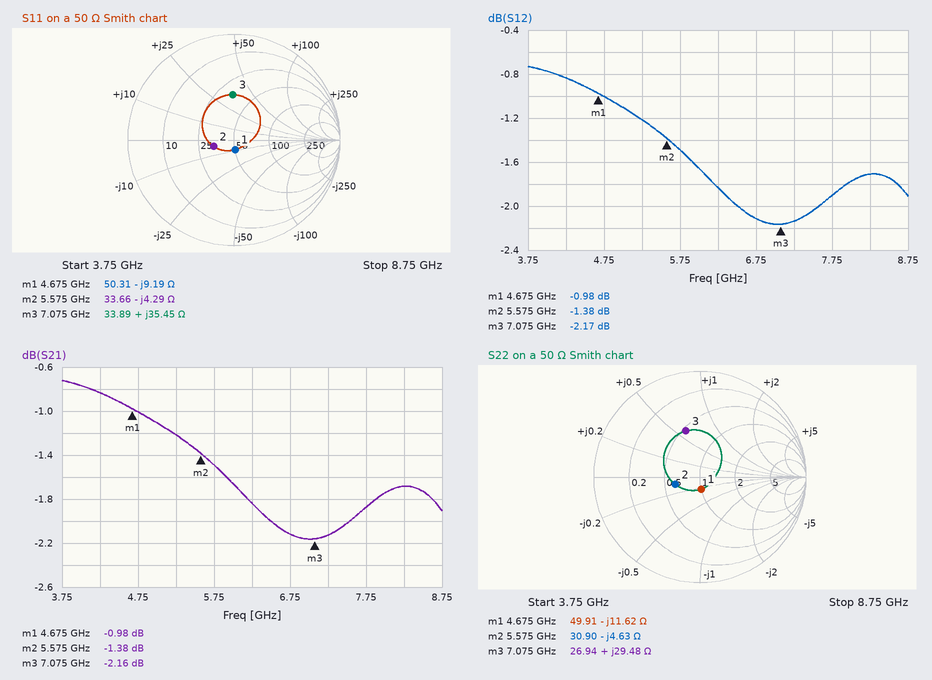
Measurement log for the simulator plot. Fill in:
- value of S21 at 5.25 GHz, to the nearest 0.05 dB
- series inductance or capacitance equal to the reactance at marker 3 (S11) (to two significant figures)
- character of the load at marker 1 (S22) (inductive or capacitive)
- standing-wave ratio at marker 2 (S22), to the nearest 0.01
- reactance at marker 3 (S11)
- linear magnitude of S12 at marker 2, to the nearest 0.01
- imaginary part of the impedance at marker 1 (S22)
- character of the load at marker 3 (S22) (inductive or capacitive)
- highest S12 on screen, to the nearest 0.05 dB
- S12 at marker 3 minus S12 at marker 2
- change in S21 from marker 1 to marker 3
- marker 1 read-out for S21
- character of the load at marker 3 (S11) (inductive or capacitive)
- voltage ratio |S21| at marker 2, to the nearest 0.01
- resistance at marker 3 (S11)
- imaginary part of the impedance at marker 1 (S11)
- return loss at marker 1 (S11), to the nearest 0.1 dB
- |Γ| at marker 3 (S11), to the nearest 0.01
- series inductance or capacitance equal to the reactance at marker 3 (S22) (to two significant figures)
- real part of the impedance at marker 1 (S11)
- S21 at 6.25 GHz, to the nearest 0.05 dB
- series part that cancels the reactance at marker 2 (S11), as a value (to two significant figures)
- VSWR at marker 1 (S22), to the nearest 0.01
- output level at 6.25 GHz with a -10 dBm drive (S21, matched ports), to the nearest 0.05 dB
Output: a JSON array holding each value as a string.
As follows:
["-1.20 dB", "800 pH", "capacitive", "1.64", "+35.45 Ω", "0.85", "-11.62 Ω", "inductive", "-0.75 dB", "-0.79 dB", "-1.18 dB", "-0.98 dB", "inductive", "0.85", "33.89 Ω", "-9.19 Ω", "20.8 dB", "0.43", "660 pH", "50.31 Ω", "-1.85 dB", "120 pH", "1.26", "-11.85 dBm"]
